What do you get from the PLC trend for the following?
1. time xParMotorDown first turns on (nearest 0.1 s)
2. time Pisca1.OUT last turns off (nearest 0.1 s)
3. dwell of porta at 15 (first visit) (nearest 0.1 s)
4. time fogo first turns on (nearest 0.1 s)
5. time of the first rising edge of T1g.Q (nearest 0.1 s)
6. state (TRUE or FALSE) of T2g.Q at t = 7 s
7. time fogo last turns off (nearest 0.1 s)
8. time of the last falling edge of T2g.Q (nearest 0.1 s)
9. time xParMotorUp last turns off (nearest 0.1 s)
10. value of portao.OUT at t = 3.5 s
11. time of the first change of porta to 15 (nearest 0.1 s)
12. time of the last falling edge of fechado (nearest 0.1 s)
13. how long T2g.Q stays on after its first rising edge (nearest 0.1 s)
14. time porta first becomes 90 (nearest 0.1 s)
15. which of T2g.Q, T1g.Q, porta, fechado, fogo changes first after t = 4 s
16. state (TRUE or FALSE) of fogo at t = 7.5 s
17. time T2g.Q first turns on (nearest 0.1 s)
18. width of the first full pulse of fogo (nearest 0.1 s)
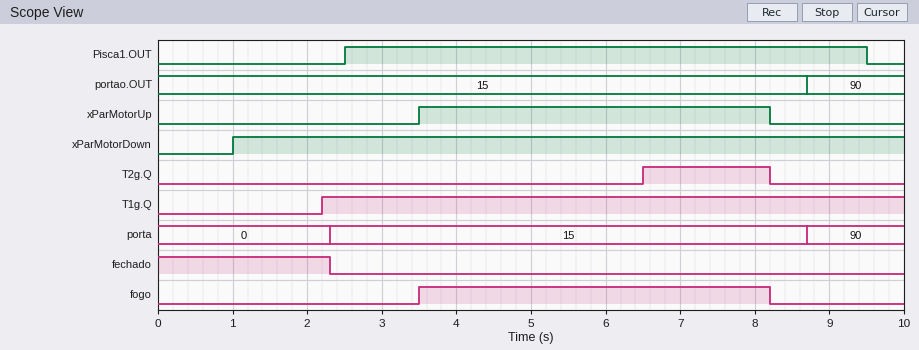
1.0 s
9.5 s
6.4 s
3.5 s
2.2 s
TRUE
8.2 s
8.2 s
8.2 s
15
2.3 s
2.3 s
1.7 s
8.7 s
T2g.Q
TRUE
6.5 s
4.7 s
